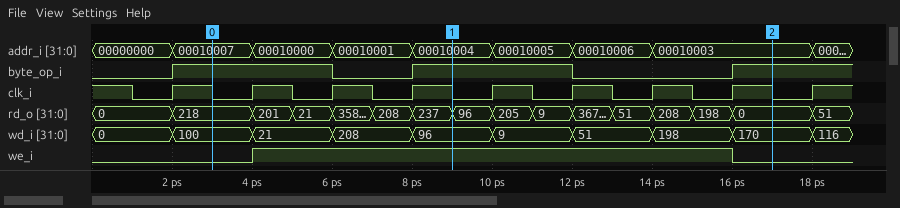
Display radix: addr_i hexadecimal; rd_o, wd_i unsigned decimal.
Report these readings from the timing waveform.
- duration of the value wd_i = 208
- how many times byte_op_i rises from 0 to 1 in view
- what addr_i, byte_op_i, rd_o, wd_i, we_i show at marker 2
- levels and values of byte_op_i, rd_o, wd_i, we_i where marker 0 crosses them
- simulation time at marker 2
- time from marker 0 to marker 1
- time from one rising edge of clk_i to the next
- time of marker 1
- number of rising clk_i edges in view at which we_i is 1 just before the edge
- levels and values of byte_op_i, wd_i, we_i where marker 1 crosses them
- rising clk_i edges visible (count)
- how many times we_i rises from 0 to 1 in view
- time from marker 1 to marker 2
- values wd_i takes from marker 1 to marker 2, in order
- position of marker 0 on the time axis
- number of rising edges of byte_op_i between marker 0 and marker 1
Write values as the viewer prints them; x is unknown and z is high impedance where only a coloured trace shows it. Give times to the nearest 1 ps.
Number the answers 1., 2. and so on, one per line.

1. 2 ps
2. 3
3. addr_i=00010003, byte_op_i=1, rd_o=0, wd_i=170, we_i=0
4. byte_op_i=1, rd_o=218, wd_i=100, we_i=0
5. 17 ps
6. 6 ps
7. 2 ps
8. 9 ps
9. 6
10. byte_op_i=1, wd_i=96, we_i=1
11. 9
12. 1
13. 8 ps
14. 96, 9, 51, 198, 170
15. 3 ps
16. 1
